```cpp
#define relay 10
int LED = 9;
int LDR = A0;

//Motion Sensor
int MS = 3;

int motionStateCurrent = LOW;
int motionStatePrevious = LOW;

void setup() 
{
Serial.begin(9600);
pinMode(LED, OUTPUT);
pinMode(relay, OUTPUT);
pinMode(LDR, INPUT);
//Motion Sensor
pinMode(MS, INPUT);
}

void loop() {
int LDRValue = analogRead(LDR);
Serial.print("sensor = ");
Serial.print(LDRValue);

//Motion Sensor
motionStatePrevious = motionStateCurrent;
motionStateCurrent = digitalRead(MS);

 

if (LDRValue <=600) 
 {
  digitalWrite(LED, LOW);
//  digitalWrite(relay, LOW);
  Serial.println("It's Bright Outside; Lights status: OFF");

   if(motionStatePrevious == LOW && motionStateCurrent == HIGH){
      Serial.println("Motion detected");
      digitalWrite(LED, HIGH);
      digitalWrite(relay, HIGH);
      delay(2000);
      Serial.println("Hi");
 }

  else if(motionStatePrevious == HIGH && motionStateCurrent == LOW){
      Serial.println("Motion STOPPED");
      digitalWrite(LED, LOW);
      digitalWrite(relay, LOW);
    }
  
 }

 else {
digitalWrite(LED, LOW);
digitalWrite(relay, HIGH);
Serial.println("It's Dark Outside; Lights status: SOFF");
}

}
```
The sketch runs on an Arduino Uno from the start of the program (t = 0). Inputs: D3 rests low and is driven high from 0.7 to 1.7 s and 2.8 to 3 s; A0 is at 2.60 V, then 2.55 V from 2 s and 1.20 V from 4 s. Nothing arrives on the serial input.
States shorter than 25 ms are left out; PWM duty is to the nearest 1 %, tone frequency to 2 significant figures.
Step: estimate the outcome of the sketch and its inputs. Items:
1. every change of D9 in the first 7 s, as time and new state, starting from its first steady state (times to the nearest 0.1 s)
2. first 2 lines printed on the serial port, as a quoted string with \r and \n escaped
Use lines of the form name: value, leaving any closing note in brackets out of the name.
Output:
every change of D9 in the first 7 s, as time and new state, starting from its first steady state: 0 s low; 0.8 s high; 2.8 s low; 2.9 s high; 4.9 s low
first 2 lines printed on the serial port, as a quoted string with \r and \n escaped: "sensor = 532It's Bright Outside; Lights status: OFF\r\nsensor = 532It's Bright Outside; Lights status: OFF\r\n"
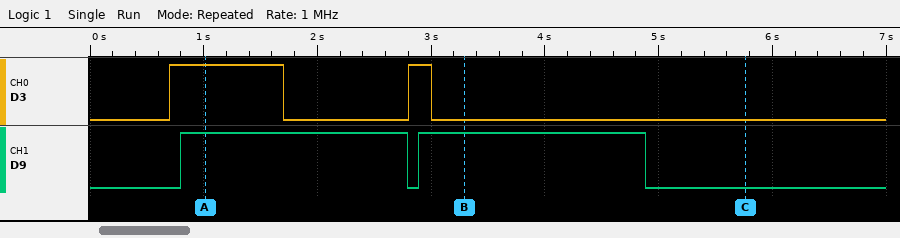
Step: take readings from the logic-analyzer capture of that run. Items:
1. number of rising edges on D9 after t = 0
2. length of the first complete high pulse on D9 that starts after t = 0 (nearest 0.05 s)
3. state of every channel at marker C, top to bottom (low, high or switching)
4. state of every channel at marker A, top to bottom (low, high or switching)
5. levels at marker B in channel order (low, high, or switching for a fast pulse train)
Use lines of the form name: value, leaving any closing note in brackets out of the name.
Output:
number of rising edges on D9 after t = 0: 2
length of the first complete high pulse on D9 that starts after t = 0: 2.00 s
state of every channel at marker C, top to bottom: D3 low, D9 low
state of every channel at marker A, top to bottom: D3 high, D9 high
levels at marker B in channel order: D3 low, D9 high
